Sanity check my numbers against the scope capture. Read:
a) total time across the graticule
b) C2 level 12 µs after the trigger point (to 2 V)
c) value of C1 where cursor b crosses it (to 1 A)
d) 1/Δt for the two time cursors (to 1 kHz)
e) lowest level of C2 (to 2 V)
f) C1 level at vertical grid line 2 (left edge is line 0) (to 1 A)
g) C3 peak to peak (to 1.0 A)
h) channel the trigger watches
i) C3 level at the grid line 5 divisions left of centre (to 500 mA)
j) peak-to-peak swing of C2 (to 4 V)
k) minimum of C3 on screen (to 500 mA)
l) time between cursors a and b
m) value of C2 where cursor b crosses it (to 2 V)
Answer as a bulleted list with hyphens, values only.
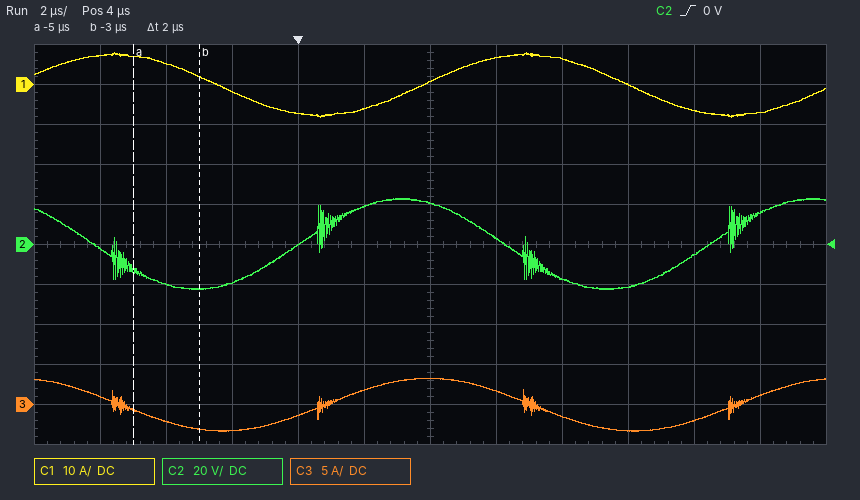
- 24 µs
- -6 V
- 2 A
- 500 kHz
- -22 V
- 5 A
- 7.0 A
- C2
- 1.0 A
- 44 V
- -3.5 A
- 2 µs
- -22 V
